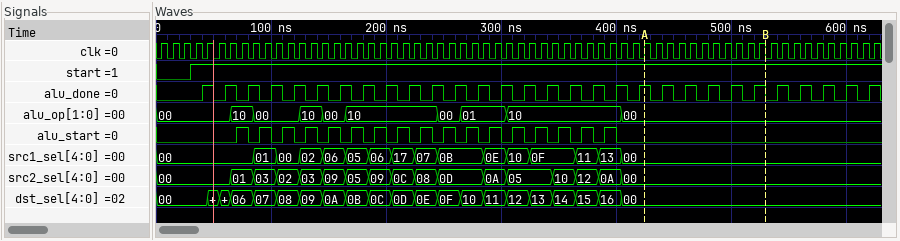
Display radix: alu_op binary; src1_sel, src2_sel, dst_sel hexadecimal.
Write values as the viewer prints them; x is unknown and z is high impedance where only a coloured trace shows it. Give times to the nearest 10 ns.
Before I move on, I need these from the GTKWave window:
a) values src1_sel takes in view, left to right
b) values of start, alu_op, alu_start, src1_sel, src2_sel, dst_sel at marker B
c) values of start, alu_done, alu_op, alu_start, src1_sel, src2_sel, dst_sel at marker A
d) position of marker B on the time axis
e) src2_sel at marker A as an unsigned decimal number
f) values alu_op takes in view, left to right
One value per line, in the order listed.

00, 01, 00, 02, 06, 05, 06, 17, 07, 0B, 0E, 10, 0F, 11, 13, 00
start=1, alu_op=00, alu_start=0, src1_sel=00, src2_sel=00, dst_sel=00
start=1, alu_done=1, alu_op=00, alu_start=0, src1_sel=00, src2_sel=00, dst_sel=00
530 ns
0
00, 10, 00, 10, 00, 10, 00, 01, 10, 00
